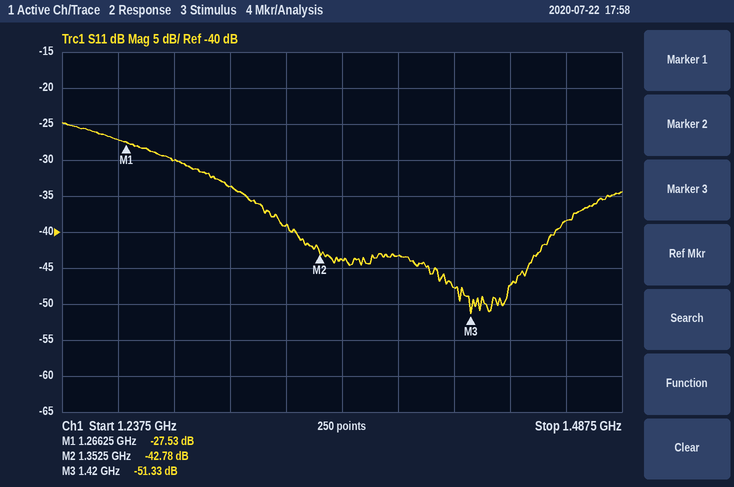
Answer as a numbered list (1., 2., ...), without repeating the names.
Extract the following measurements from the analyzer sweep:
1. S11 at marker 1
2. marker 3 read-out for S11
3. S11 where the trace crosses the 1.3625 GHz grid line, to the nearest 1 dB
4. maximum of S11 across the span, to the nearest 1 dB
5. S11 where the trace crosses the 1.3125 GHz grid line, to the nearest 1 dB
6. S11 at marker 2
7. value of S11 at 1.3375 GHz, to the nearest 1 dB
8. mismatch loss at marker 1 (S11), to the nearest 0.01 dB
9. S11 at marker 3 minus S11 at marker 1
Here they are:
1. -27.53 dB
2. -51.33 dB
3. -44 dB
4. -25 dB
5. -34 dB
6. -42.78 dB
7. -39 dB
8. 0.01 dB
9. -23.80 dB
